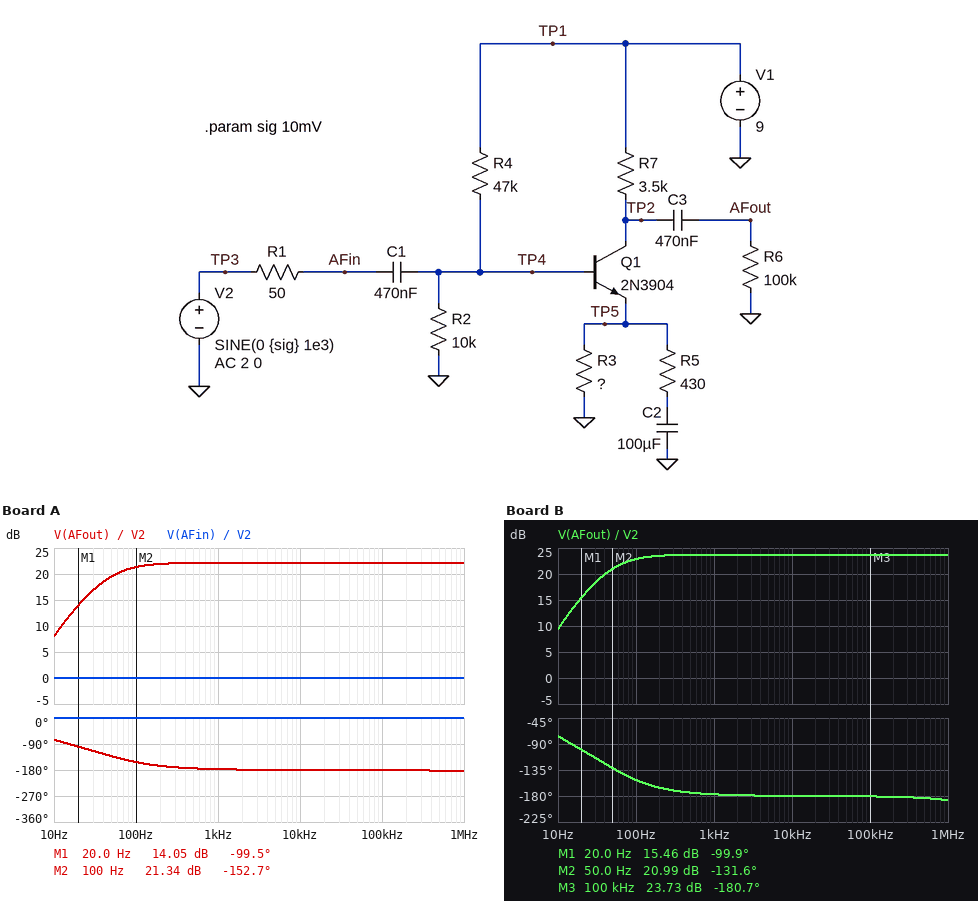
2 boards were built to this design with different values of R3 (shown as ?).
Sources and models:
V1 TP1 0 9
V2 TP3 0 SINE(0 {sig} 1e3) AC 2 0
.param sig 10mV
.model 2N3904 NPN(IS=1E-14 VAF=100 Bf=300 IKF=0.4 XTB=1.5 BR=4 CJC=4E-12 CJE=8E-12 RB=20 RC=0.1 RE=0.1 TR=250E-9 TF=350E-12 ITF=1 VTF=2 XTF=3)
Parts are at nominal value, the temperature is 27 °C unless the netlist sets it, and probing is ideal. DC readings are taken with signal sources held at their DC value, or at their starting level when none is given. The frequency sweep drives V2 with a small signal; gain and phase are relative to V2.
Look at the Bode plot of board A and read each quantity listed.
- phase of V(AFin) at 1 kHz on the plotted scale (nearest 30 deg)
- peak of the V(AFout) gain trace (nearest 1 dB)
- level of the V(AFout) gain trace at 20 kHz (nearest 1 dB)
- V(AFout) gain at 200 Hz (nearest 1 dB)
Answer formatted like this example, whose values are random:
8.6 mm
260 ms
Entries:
0 deg
22 dB
22 dB
22 dB
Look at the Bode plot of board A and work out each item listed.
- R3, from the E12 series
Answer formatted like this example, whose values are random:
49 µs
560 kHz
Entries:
560 Ω
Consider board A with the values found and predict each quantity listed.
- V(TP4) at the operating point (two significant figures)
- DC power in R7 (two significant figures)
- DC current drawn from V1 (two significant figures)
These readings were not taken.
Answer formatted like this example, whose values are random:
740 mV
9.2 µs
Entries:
1.5 V
8.4 mW
1.7 mA
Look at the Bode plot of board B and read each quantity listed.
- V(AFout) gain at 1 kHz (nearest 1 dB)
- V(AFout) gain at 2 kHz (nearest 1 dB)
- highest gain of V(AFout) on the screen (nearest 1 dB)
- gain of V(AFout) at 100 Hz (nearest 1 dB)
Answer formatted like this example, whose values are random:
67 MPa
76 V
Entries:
24 dB
24 dB
24 dB
23 dB
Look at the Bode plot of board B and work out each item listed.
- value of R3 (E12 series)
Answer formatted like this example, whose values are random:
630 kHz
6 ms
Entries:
390 Ω
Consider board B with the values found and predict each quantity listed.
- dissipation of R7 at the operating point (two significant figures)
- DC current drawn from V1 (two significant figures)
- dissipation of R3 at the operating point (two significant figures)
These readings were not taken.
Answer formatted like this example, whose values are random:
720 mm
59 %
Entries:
16 mW
2.3 mA
1.8 mW
